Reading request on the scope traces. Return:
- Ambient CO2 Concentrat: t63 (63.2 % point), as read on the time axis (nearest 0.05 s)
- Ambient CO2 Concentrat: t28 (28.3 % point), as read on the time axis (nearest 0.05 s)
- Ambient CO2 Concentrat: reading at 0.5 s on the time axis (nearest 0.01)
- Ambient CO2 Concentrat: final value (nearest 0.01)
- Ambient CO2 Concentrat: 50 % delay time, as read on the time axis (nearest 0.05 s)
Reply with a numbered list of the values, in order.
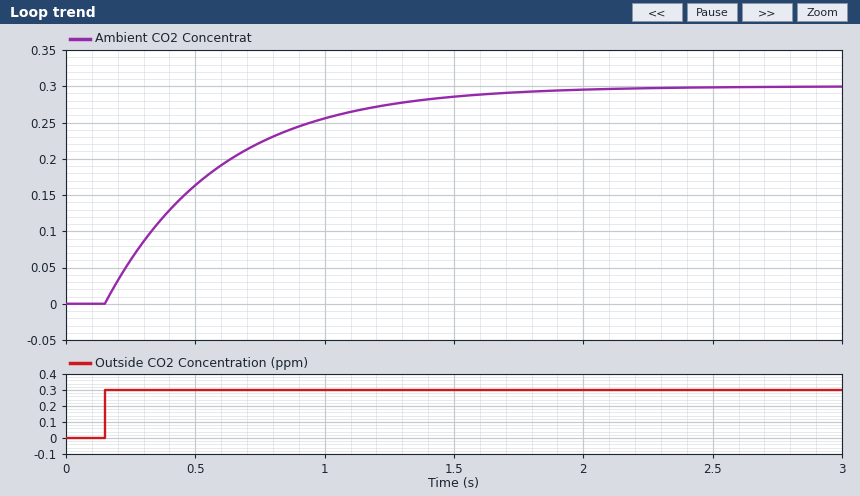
1. 0.60 s
2. 0.30 s
3. 0.16
4. 0.30
5. 0.45 s
